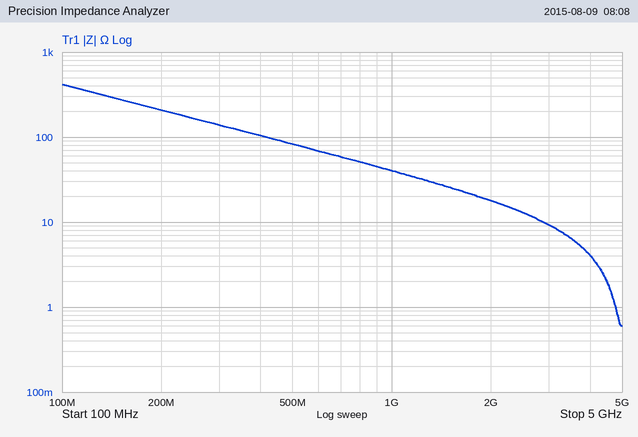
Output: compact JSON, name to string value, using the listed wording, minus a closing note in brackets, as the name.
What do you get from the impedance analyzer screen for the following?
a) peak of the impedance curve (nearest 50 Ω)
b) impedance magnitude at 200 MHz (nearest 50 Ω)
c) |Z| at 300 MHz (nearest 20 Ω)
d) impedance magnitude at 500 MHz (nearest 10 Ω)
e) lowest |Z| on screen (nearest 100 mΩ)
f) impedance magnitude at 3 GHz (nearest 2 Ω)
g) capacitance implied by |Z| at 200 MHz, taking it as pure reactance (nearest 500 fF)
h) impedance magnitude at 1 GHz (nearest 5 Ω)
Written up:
{"peak of the impedance curve": "400 Ω", "impedance magnitude at 200 MHz": "200 Ω", "|Z| at 300 MHz": "140 Ω", "impedance magnitude at 500 MHz": "80 Ω", "lowest |Z| on screen": "600 mΩ", "impedance magnitude at 3 GHz": "10 Ω", "capacitance implied by |Z| at 200 MHz, taking it as pure reactance": "4.0 pF", "impedance magnitude at 1 GHz": "40 Ω"}
